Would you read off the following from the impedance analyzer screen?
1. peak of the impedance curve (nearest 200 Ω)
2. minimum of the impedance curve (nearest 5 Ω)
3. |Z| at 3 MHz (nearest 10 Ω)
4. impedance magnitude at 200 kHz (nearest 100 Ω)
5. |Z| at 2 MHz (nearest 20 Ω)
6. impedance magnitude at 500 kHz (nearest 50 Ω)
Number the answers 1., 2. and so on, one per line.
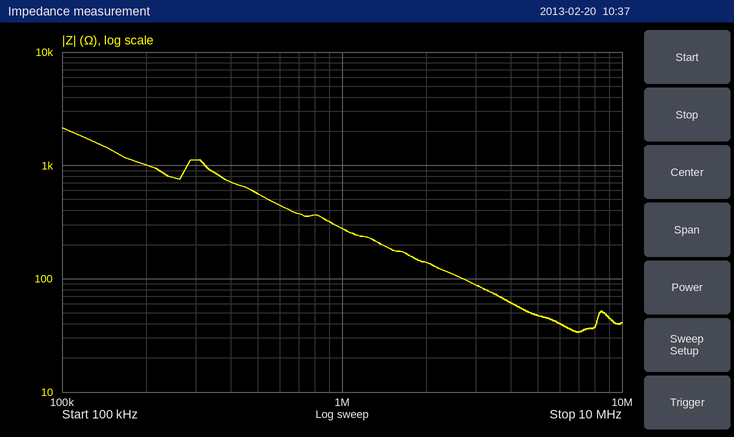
1. 2.2 kΩ
2. 35 Ω
3. 90 Ω
4. 1.0 kΩ
5. 140 Ω
6. 550 Ω
